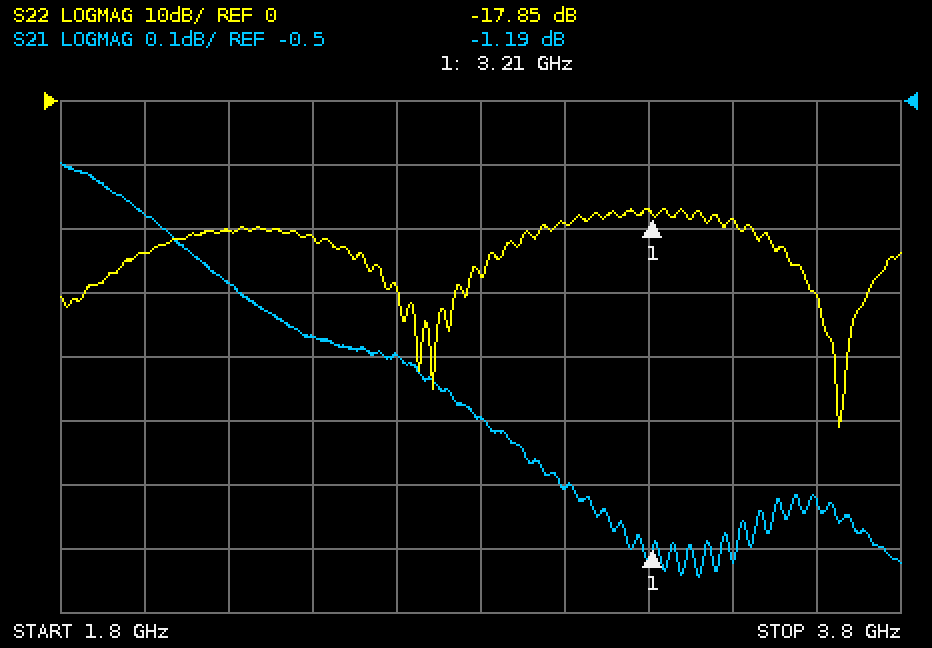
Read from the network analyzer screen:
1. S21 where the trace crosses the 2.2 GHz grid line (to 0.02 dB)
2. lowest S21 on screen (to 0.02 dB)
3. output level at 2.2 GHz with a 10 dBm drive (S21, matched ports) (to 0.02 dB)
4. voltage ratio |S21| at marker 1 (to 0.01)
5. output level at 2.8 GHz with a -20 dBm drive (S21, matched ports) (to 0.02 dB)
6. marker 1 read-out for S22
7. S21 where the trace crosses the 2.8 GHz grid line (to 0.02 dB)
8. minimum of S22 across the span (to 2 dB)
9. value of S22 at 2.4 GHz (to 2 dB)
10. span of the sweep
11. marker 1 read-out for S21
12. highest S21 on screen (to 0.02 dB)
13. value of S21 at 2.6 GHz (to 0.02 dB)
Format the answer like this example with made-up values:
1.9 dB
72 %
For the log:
-0.78 dB
-1.24 dB
9.22 dBm
0.87
-21.00 dBm
-17.85 dB
-1.00 dB
-50 dB
-22 dB
2 GHz
-1.19 dB
-0.60 dB
-0.90 dB
